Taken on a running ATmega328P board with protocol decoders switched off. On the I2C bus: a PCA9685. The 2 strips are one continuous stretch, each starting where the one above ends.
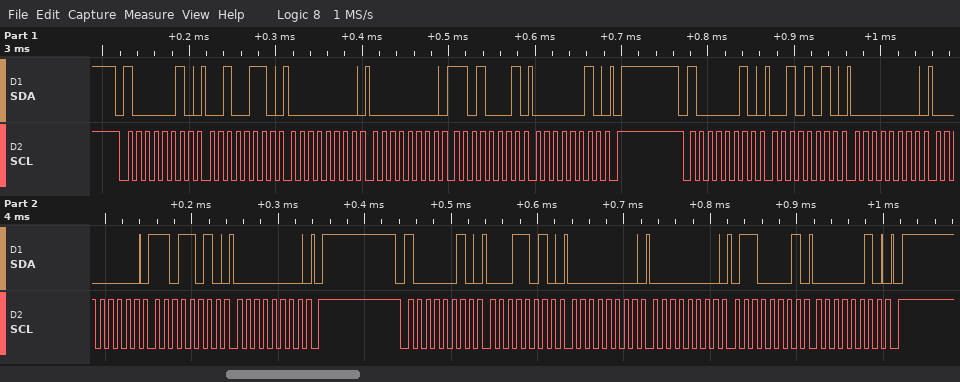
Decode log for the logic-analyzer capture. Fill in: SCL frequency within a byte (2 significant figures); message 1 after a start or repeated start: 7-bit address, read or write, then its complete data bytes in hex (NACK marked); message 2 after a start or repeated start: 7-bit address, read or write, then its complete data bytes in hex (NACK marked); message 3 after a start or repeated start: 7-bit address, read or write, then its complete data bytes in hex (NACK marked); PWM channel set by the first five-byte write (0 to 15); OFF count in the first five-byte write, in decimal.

100 kHz
0x41 write: 26 00 00 D1 02
0x41 write: 2A 00 00 DA 00
0x41 write: 1A 00 00 61 02
8
721
